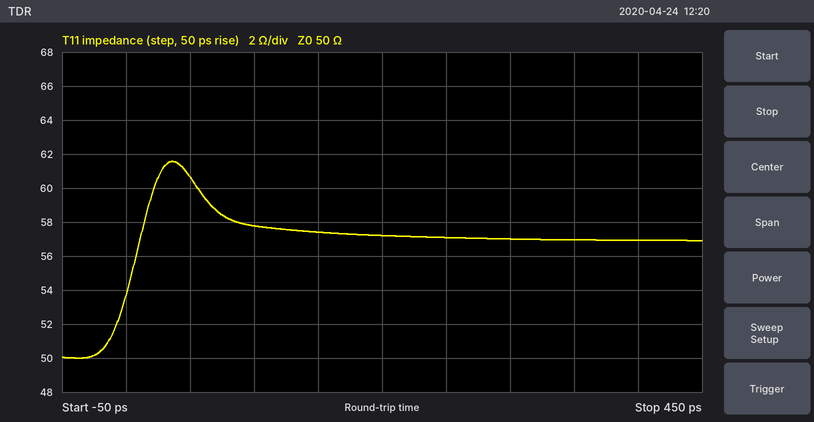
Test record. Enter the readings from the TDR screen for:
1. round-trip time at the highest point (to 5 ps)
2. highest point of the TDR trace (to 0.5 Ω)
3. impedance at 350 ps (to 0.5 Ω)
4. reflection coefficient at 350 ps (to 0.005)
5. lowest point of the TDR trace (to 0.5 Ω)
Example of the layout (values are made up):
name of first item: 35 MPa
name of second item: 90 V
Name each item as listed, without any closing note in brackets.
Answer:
round-trip time at the highest point: 35 ps
highest point of the TDR trace: 61.5 Ω
impedance at 350 ps: 57.0 Ω
reflection coefficient at 350 ps: +0.065
lowest point of the TDR trace: 50.0 Ω
